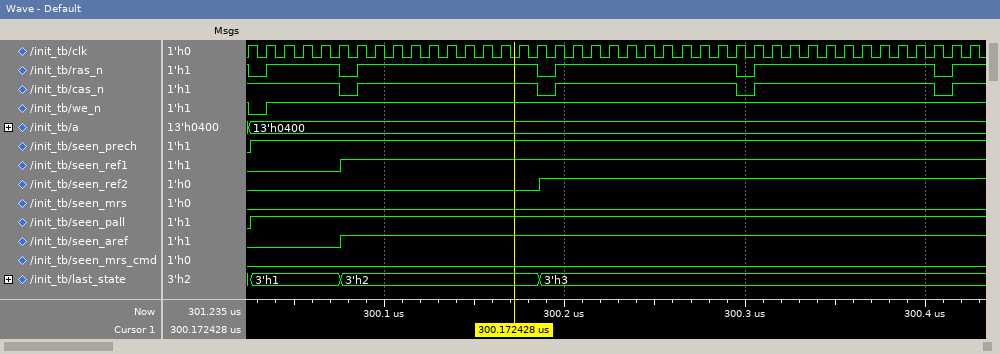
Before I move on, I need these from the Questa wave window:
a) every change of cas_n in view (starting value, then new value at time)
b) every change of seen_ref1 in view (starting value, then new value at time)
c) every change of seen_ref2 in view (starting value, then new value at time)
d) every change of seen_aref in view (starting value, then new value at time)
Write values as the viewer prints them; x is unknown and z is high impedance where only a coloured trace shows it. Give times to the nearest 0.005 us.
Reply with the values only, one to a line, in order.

1, 0 at 300.075 us, 1 at 300.085 us, 0 at 300.185 us, 1 at 300.195 us, 0 at 300.295 us, 1 at 300.305 us, 0 at 300.405 us, 1 at 300.415 us
0, 1 at 300.075 us
0, 1 at 300.185 us
0, 1 at 300.075 us
